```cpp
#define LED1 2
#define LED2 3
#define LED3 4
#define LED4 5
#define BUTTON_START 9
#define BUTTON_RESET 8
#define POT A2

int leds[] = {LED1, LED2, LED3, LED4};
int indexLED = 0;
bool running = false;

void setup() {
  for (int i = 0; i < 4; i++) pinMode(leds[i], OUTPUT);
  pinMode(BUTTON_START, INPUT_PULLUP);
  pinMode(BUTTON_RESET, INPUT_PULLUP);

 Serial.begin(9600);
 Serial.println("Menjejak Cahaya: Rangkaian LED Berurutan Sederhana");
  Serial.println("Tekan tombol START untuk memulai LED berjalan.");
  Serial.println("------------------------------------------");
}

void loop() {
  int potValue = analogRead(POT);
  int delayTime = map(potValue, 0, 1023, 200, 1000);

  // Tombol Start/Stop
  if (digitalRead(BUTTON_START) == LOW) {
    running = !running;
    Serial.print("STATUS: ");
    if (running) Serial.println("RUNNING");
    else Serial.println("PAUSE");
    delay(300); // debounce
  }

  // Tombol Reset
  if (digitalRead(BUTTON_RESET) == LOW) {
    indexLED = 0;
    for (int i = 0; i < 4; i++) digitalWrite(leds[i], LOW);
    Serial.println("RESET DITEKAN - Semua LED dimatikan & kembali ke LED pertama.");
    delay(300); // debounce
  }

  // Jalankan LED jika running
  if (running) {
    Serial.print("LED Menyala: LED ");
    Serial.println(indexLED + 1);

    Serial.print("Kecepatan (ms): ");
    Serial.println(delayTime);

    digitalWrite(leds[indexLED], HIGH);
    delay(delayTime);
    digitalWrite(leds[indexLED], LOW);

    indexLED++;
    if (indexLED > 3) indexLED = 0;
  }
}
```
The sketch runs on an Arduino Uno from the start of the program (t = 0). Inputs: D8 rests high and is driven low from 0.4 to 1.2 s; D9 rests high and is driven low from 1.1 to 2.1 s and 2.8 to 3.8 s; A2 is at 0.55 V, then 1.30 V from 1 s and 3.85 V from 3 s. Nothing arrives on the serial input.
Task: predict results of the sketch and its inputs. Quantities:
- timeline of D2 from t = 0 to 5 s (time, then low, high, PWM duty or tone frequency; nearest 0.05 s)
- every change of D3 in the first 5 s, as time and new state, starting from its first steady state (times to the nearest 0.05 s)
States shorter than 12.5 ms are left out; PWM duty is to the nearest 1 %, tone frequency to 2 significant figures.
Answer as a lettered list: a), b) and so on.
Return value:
a) 0 s low; 1.6 s high; 2 s low
b) 0 s low; 3.1 s high; 3.5 s low
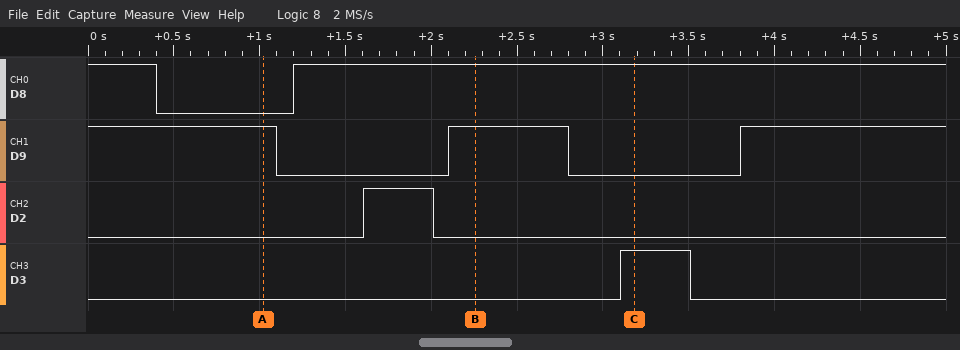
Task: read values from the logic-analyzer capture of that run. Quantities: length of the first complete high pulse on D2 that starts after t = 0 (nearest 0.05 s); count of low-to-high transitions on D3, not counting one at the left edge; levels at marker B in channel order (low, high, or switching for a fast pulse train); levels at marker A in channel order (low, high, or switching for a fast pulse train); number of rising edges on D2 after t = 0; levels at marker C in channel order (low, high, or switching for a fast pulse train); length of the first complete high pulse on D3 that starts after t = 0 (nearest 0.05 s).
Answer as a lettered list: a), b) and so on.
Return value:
a) 0.40 s
b) 1
c) D8 high, D9 high, D2 low, D3 low
d) D8 low, D9 high, D2 low, D3 low
e) 1
f) D8 high, D9 low, D2 low, D3 high
g) 0.40 s
